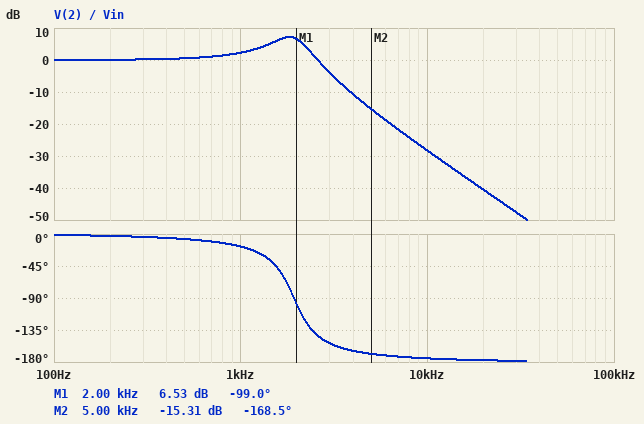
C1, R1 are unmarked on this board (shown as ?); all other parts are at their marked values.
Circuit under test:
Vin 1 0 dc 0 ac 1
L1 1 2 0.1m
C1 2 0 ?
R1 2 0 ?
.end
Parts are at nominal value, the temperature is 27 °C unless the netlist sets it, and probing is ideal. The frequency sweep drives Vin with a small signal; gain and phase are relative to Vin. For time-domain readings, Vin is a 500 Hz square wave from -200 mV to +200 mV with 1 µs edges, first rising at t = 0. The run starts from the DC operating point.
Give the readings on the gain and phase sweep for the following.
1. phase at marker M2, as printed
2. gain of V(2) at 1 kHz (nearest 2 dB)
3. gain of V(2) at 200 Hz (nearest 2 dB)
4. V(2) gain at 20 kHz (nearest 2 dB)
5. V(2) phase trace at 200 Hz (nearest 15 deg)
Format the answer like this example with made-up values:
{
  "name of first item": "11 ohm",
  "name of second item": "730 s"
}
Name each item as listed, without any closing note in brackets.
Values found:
{
  "phase at marker M2, as printed": "-168.5 deg",
  "gain of V(2) at 1 kHz": "2 dB",
  "gain of V(2) at 200 Hz": "0 dB",
  "V(2) gain at 20 kHz": "-40 dB",
  "V(2) phase trace at 200 Hz": "0 deg"
}
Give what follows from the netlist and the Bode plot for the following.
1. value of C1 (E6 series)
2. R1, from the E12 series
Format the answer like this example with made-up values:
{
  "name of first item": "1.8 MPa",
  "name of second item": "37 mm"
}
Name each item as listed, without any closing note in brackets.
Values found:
{
  "value of C1": "68 µF",
  "R1, from the E12 series": "2.7 Ω"
}
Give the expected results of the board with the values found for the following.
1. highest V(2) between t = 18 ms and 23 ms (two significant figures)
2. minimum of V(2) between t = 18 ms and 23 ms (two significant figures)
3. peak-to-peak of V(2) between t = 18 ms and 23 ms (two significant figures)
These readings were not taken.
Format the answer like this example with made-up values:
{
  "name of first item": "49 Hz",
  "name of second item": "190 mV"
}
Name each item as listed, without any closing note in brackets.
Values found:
{
  "highest V(2) between t = 18 ms and 23 ms": "390 mV",
  "minimum of V(2) between t = 18 ms and 23 ms": "-390 mV",
  "peak-to-peak of V(2) between t = 18 ms and 23 ms": "770 mV"
}
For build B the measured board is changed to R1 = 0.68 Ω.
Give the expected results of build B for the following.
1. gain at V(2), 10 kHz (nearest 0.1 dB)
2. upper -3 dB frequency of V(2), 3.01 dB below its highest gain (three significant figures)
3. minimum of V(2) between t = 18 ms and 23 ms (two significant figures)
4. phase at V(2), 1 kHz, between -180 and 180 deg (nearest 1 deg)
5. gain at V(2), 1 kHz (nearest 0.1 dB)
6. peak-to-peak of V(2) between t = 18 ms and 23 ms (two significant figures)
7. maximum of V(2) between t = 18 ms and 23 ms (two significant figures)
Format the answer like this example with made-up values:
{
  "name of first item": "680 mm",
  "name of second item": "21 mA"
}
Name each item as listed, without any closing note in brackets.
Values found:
{
  "gain at V(2), 10 kHz": "-28.8 dB",
  "upper -3 dB frequency of V(2), 3.01 dB below its highest gain": "1.46 kHz",
  "minimum of V(2) between t = 18 ms and 23 ms": "-200 mV",
  "phase at V(2), 1 kHz, between -180 and 180 deg": "-52 deg",
  "gain at V(2), 1 kHz": "-1.4 dB",
  "peak-to-peak of V(2) between t = 18 ms and 23 ms": "400 mV",
  "maximum of V(2) between t = 18 ms and 23 ms": "200 mV"
}
